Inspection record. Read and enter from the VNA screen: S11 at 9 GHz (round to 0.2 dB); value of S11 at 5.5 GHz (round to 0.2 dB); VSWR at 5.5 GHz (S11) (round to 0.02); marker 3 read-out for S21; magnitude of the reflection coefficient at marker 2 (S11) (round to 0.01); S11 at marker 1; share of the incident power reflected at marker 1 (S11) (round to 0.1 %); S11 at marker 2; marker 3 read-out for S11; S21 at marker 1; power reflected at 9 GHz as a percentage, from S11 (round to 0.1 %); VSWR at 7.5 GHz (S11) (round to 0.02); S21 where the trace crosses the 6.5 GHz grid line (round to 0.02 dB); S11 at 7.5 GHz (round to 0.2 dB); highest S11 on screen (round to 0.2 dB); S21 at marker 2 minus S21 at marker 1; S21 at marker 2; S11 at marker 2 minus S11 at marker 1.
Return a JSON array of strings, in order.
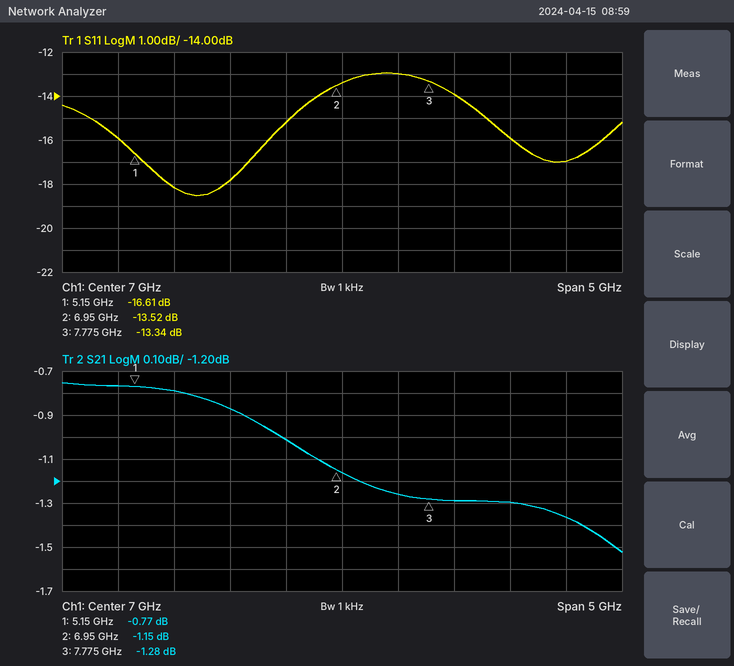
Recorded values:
["-17.0 dB", "-18.2 dB", "1.28", "-1.28 dB", "0.21", "-16.61 dB", "2.2 %", "-13.52 dB", "-13.34 dB", "-0.77 dB", "2.0 %", "1.58", "-1.02 dB", "-13.0 dB", "-13.0 dB", "-0.38 dB", "-1.15 dB", "3.09 dB"]
